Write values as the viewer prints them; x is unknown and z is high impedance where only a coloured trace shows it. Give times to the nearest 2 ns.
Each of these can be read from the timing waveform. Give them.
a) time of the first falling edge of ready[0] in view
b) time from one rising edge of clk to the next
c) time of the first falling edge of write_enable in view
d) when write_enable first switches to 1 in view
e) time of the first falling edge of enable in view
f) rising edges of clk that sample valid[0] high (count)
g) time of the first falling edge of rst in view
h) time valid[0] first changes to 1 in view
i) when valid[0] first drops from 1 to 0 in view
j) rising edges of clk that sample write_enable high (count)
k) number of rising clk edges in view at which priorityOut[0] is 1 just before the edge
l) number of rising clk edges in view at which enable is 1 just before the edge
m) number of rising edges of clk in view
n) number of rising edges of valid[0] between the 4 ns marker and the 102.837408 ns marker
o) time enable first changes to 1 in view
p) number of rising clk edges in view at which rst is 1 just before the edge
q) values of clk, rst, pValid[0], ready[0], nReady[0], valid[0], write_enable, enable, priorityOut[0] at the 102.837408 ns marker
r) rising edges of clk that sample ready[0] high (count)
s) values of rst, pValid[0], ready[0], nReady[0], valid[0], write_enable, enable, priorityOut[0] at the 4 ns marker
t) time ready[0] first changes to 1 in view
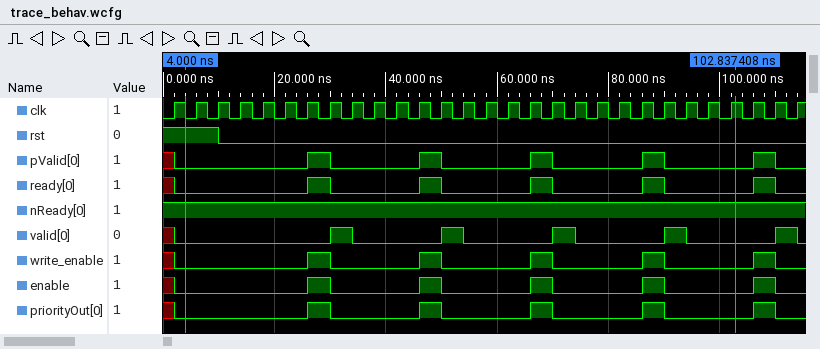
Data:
30 ns
4 ns
30 ns
26 ns
30 ns
5
10 ns
30 ns
34 ns
5
5
5
29
4
26 ns
3
clk=1, rst=0, pValid[0]=0, ready[0]=0, nReady[0]=1, valid[0]=0, write_enable=0, enable=0, priorityOut[0]=0
5
rst=1, pValid[0]=0, ready[0]=0, nReady[0]=1, valid[0]=0, write_enable=0, enable=0, priorityOut[0]=0
26 ns
